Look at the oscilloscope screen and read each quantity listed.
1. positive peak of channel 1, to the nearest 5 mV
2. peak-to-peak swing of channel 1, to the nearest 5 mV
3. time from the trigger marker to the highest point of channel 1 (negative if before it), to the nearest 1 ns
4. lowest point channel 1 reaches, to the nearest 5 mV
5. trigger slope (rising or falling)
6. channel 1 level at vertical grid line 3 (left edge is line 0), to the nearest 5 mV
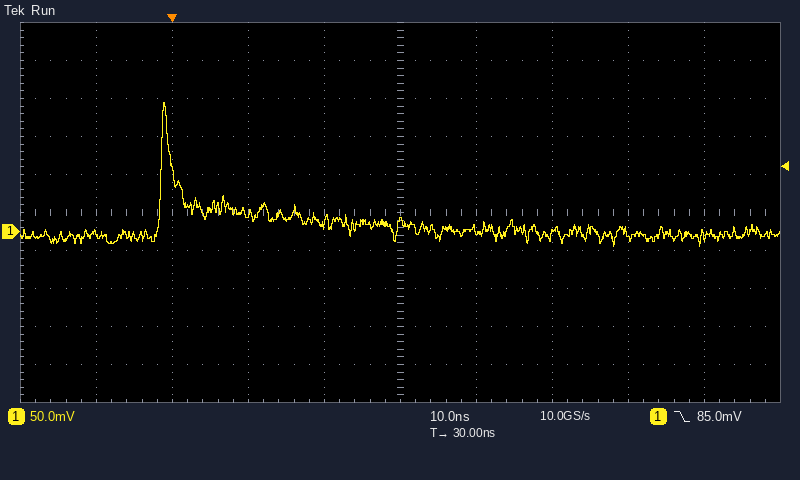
170 mV
190 mV
-1 ns
-20 mV
falling
25 mV
